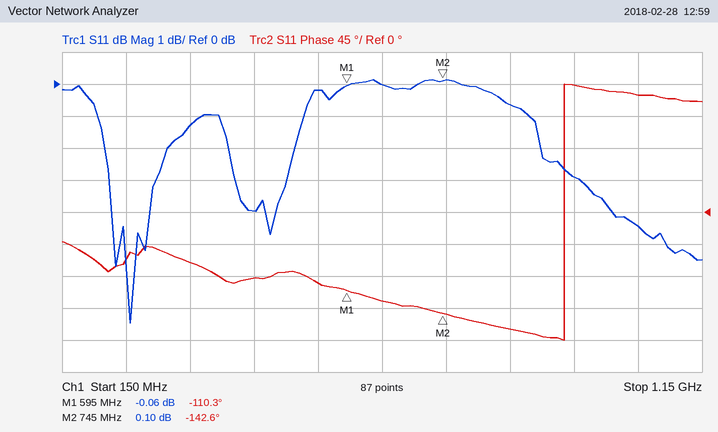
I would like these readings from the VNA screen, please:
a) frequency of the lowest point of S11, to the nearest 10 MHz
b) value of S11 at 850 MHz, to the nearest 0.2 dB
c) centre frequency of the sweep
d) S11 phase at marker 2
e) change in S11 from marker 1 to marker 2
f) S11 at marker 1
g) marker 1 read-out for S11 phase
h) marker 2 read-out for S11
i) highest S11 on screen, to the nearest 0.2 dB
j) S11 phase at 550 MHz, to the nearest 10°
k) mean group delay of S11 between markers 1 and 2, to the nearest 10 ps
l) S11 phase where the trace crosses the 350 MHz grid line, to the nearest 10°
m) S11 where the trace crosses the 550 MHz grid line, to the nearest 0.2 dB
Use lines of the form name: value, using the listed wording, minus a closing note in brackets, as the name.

frequency of the lowest point of S11, to the nearest 10 MHz: 260 MHz
value of S11 at 850 MHz, to the nearest 0.2 dB: -0.6 dB
centre frequency of the sweep: 650 MHz
S11 phase at marker 2: -142.6°
change in S11 from marker 1 to marker 2: 0.16 dB
S11 at marker 1: -0.06 dB
marker 1 read-out for S11 phase: -110.3°
marker 2 read-out for S11: 0.10 dB
highest S11 on screen, to the nearest 0.2 dB: 0.2 dB
S11 phase at 550 MHz, to the nearest 10°: -100°
mean group delay of S11 between markers 1 and 2, to the nearest 10 ps: 600 ps
S11 phase where the trace crosses the 350 MHz grid line, to the nearest 10°: -70°
S11 where the trace crosses the 550 MHz grid line, to the nearest 0.2 dB: -0.2 dB
